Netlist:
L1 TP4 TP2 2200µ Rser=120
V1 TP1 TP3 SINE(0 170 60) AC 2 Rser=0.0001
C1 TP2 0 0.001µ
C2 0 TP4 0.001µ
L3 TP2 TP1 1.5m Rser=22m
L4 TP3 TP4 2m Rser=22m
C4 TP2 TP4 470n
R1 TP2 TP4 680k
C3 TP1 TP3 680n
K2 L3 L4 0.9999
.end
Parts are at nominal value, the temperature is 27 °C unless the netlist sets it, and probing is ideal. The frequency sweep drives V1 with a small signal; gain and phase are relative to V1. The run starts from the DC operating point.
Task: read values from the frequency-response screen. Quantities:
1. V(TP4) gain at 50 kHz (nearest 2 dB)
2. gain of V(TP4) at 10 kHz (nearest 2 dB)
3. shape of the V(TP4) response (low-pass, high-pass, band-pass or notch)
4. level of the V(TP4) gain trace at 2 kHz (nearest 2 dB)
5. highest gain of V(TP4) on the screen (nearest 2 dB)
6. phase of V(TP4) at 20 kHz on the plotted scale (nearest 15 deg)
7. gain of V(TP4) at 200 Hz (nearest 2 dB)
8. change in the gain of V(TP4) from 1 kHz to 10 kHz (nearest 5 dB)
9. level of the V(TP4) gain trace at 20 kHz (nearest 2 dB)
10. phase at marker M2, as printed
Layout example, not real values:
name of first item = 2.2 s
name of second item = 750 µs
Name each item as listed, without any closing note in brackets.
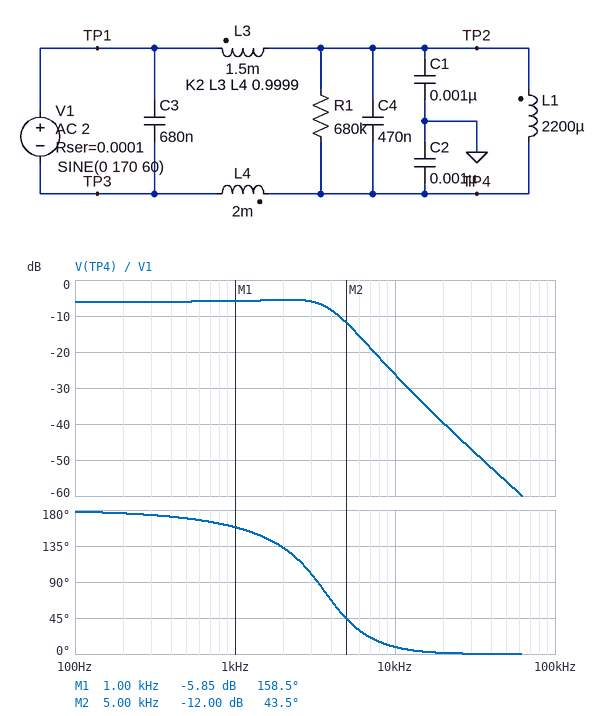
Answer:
V(TP4) gain at 50 kHz = -56 dB
gain of V(TP4) at 10 kHz = -26 dB
shape of the V(TP4) response = low-pass
level of the V(TP4) gain trace at 2 kHz = -6 dB
highest gain of V(TP4) on the screen = -6 dB
phase of V(TP4) at 20 kHz on the plotted scale = 0 deg
gain of V(TP4) at 200 Hz = -6 dB
change in the gain of V(TP4) from 1 kHz to 10 kHz = -20 dB
level of the V(TP4) gain trace at 20 kHz = -40 dB
phase at marker M2, as printed = 43.5 deg
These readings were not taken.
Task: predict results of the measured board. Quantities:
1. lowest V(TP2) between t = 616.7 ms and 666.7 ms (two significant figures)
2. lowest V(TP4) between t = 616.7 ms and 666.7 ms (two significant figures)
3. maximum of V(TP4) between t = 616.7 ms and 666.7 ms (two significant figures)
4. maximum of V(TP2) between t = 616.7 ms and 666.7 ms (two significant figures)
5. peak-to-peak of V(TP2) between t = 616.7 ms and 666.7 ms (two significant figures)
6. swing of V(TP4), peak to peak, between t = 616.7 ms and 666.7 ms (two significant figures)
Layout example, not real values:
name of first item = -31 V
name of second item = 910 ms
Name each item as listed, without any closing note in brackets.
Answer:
lowest V(TP2) between t = 616.7 ms and 666.7 ms = -85 V
lowest V(TP4) between t = 616.7 ms and 666.7 ms = -85 V
maximum of V(TP4) between t = 616.7 ms and 666.7 ms = 85 V
maximum of V(TP2) between t = 616.7 ms and 666.7 ms = 85 V
peak-to-peak of V(TP2) between t = 616.7 ms and 666.7 ms = 170 V
swing of V(TP4), peak to peak, between t = 616.7 ms and 666.7 ms = 170 V
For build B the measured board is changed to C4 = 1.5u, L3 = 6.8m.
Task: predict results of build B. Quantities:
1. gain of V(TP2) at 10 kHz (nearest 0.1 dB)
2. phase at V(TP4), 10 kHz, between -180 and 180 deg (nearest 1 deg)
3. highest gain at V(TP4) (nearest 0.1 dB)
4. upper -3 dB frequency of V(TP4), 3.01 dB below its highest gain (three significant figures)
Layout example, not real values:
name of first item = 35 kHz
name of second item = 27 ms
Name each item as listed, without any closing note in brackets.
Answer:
gain of V(TP2) at 10 kHz = -45.2 dB
phase at V(TP4), 10 kHz, between -180 and 180 deg = 2 deg
highest gain at V(TP4) = -4.2 dB
upper -3 dB frequency of V(TP4), 3.01 dB below its highest gain = 1.28 kHz
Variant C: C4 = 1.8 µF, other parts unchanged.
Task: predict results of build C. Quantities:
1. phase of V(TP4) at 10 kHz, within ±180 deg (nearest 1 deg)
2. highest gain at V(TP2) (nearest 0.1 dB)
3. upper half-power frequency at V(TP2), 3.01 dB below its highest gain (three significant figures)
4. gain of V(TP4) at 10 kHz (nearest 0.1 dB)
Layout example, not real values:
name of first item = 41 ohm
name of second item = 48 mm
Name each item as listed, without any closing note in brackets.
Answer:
phase of V(TP4) at 10 kHz, within ±180 deg = 2 deg
highest gain at V(TP2) = -0.2 dB
upper half-power frequency at V(TP2), 3.01 dB below its highest gain = 1.74 kHz
gain of V(TP4) at 10 kHz = -39.4 dB
